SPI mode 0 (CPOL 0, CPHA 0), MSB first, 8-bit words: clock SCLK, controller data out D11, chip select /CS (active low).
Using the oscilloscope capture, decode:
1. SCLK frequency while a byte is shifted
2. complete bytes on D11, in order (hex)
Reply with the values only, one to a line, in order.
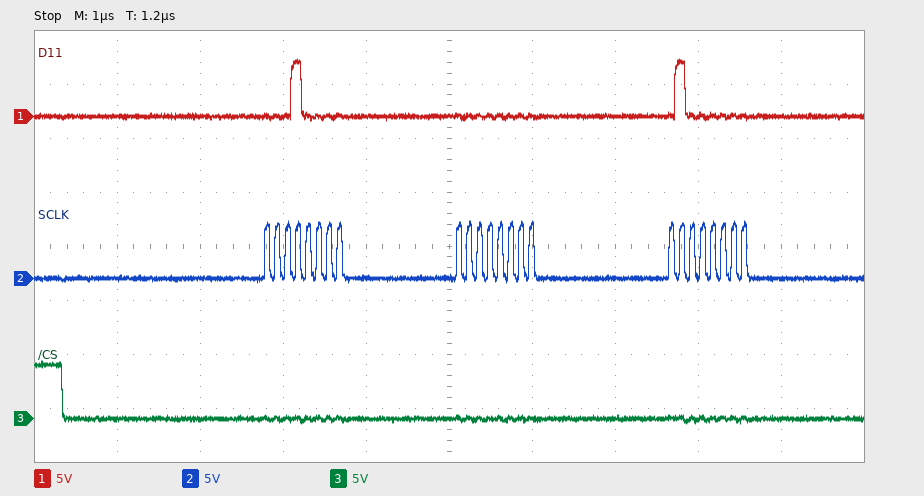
8 MHz
10 00 40
